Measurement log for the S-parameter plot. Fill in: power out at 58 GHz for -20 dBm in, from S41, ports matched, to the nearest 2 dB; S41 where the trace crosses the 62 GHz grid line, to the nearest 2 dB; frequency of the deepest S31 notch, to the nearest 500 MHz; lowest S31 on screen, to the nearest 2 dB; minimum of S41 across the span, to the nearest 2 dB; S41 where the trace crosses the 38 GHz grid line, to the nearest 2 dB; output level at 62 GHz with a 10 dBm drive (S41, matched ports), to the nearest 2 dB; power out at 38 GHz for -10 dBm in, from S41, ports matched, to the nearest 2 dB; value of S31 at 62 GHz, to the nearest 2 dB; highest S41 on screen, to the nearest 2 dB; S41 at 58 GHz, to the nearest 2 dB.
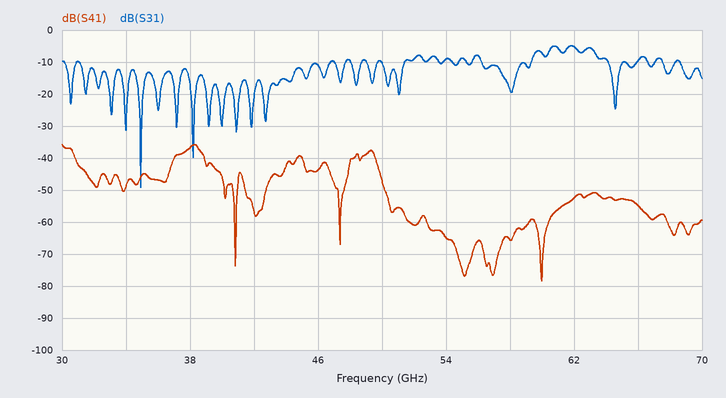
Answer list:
-86 dBm
-52 dB
35.0 GHz
-50 dB
-78 dB
-36 dB
-42 dBm
-46 dBm
-6 dB
-36 dB
-66 dB
